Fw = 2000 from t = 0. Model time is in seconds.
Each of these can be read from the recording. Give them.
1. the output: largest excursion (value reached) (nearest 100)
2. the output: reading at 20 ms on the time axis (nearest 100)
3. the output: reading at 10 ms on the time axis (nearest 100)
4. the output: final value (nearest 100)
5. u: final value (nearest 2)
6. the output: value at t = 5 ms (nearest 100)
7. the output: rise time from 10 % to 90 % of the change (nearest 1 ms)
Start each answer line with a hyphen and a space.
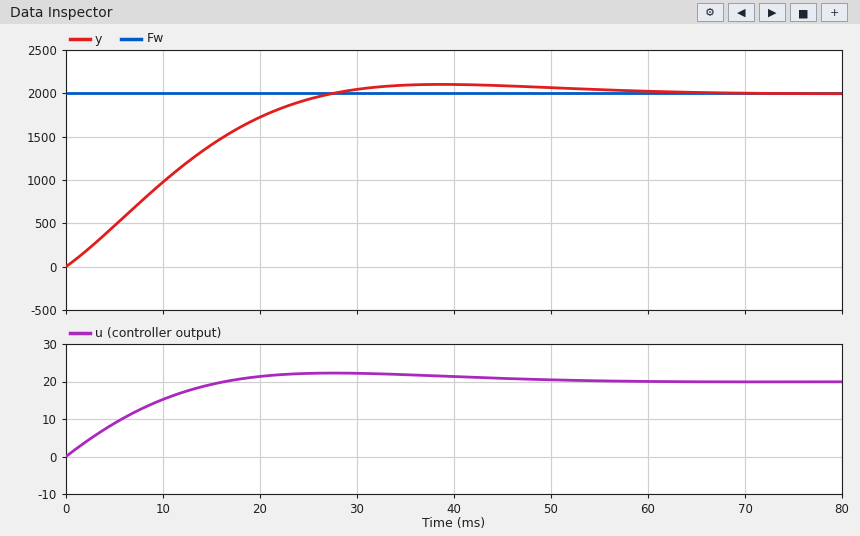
- 2100
- 1700
- 1000
- 2000
- 20
- 500
- 19 ms
